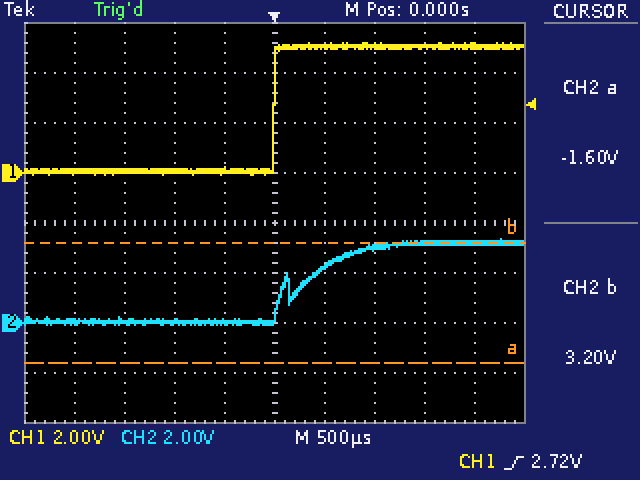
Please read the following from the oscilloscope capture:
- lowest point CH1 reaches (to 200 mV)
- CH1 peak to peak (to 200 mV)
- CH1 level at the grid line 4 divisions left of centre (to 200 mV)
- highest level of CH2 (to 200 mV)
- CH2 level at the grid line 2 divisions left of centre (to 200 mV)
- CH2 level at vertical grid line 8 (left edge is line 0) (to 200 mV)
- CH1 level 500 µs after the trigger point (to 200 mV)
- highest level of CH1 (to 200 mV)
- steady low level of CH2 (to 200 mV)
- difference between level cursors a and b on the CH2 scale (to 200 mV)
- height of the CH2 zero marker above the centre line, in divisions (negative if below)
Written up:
0.0 V
5.2 V
0.0 V
3.4 V
0.0 V
3.2 V
5.0 V
5.2 V
0.0 V
4.8 V
-2.0 div
